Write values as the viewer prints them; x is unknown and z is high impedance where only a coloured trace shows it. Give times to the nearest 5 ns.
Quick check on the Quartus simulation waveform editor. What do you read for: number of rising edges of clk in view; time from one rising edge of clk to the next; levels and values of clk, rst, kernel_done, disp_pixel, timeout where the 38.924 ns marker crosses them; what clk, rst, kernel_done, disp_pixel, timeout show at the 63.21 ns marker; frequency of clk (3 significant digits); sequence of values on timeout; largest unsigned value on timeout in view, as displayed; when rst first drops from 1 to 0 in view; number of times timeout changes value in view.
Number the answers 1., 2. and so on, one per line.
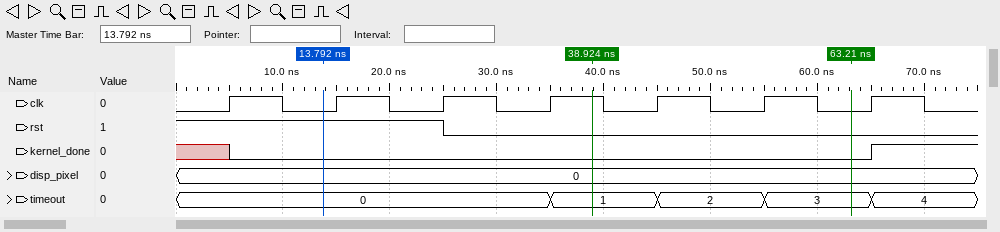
1. 7
2. 10 ns
3. clk=1, rst=0, kernel_done=0, disp_pixel=0, timeout=1
4. clk=0, rst=0, kernel_done=0, disp_pixel=0, timeout=3
5. 100 MHz
6. 0, 1, 2, 3, 4
7. 4
8. 25 ns
9. 4
